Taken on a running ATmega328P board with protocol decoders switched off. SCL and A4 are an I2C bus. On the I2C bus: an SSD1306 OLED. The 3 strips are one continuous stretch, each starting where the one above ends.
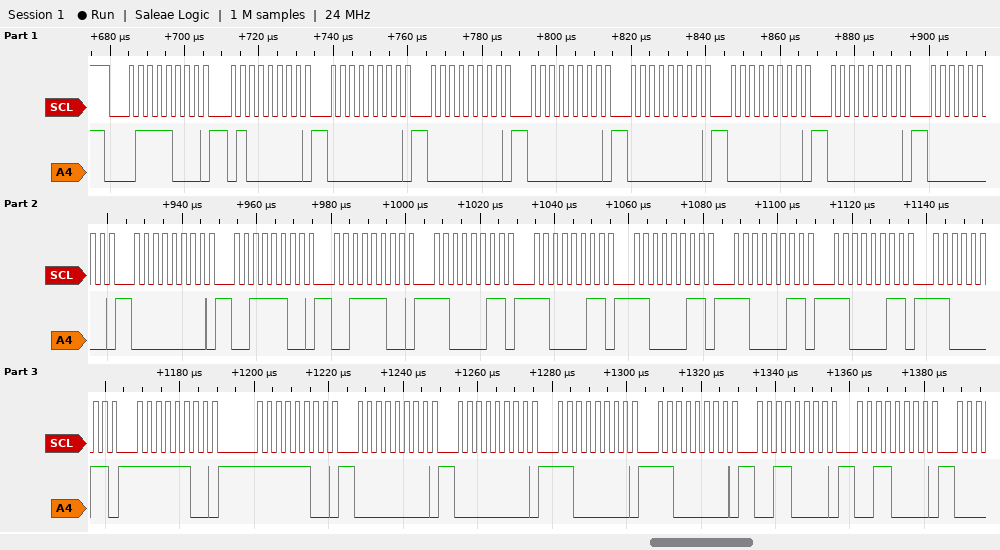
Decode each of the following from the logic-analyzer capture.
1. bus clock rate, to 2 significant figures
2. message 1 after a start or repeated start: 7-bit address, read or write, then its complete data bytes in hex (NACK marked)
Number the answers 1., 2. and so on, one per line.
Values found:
1. 400 kHz
2. 0x3C write: 40 00 00 00 00 00 00 00 00 3C 3C C3 C3 C3 C3 C3 C3 FC FC 00 00 C0 C0 30 30
